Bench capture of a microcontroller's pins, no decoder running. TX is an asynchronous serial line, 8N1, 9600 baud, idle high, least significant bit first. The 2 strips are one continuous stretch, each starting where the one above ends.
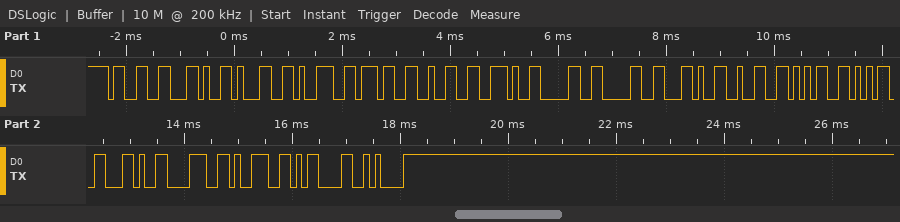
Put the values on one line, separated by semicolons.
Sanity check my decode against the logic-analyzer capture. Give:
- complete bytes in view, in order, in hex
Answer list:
0x33 0x2C 0x31 0x39 0x37 0x32 0x2E 0x30 0x30 0x2C 0x32 0x35 0x35 0x2C 0x38 0x39 0x0D 0x0A
